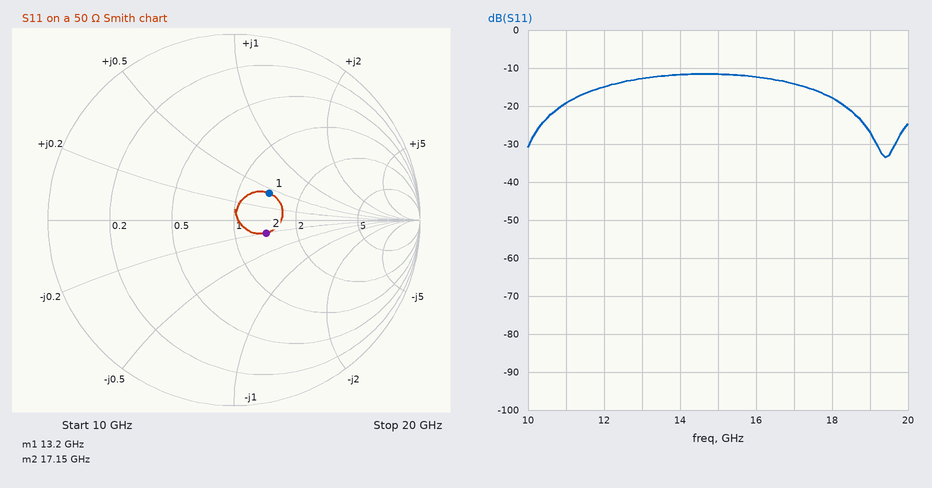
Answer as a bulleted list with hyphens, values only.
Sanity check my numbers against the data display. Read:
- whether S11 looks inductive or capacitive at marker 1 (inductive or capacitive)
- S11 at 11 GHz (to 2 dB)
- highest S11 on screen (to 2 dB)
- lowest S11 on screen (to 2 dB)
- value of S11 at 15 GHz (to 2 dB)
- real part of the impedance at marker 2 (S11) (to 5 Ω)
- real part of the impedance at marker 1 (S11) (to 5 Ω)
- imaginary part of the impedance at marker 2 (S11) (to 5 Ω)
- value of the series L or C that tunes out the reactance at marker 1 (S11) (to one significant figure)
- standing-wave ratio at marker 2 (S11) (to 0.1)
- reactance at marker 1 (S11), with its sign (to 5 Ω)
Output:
- inductive
- -20 dB
- -12 dB
- -34 dB
- -12 dB
- 70 Ω
- 70 Ω
- -10 Ω
- 600 fF
- 1.5
- +20 Ω
